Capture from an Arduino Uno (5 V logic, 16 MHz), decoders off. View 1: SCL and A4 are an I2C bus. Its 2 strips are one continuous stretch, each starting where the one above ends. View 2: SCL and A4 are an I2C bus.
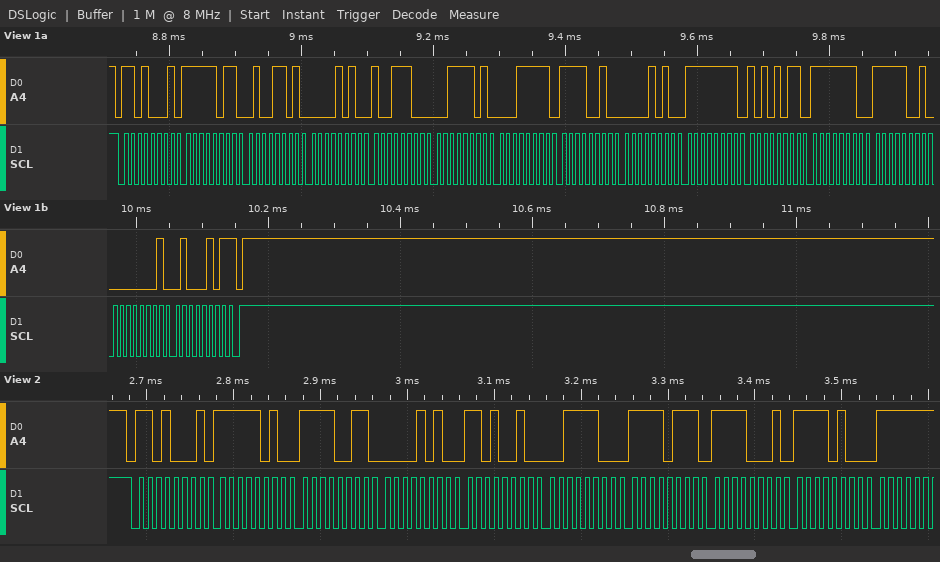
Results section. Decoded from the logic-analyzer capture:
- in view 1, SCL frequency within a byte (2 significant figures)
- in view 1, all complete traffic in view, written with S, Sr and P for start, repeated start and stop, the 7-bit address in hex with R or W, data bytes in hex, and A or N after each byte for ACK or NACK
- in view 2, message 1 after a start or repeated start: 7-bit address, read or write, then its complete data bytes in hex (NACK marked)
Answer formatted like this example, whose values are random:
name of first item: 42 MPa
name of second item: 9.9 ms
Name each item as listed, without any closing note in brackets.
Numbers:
in view 1, SCL frequency within a byte: 100 kHz
in view 1, all complete traffic in view, written with S, Sr and P for start, repeated start and stop, the 7-bit address in hex with R or W, data bytes in hex, and A or N after each byte for ACK or NACK: S 68R A FB A 4D A 0A A 9C A 3D A 1F A F2 A 0A A FF A AB A FE A F9 A 01 A 45 N P
in view 2, message 1 after a start or repeated start: 7-bit address, read or write, then its complete data bytes in hex: 0x68 read: FA F3 0A D2 3C F7 F1 F4
